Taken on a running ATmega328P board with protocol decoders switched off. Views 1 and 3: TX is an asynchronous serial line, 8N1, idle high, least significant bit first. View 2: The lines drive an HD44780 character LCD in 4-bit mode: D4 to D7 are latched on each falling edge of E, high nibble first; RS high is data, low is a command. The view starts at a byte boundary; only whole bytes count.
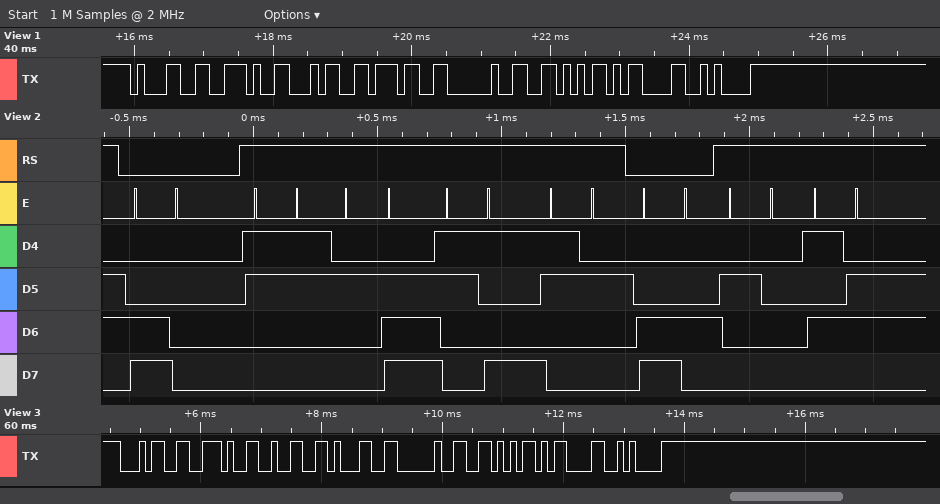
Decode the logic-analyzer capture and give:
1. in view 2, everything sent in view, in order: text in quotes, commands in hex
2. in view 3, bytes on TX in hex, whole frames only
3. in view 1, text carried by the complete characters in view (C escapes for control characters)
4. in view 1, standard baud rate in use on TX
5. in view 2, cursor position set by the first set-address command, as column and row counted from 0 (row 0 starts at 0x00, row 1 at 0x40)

0xC0 "3.92" 0xC4 " V"
0x34 0x2E 0x32 0x31 0x20 0x56 0x0D 0x0A
"1.47 V\r\n"
9600 baud
column 0, row 1
